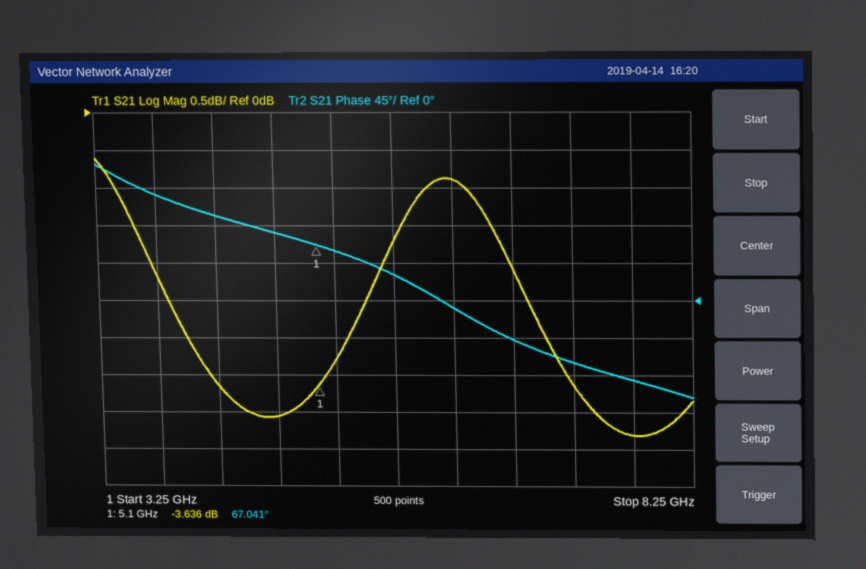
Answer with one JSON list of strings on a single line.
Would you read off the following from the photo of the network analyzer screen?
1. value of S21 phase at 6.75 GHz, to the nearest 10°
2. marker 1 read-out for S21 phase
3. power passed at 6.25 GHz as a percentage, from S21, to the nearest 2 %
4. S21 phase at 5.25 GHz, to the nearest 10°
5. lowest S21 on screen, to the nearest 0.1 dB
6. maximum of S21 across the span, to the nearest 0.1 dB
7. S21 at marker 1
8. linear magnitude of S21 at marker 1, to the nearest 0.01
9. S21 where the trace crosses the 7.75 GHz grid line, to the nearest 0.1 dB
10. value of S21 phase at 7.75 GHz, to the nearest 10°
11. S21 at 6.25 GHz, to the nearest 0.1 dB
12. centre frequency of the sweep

["-50°", "67.041°", "82 %", "60°", "-4.3 dB", "-0.6 dB", "-3.636 dB", "0.66", "-4.3 dB", "-100°", "-0.9 dB", "5.75 GHz"]
